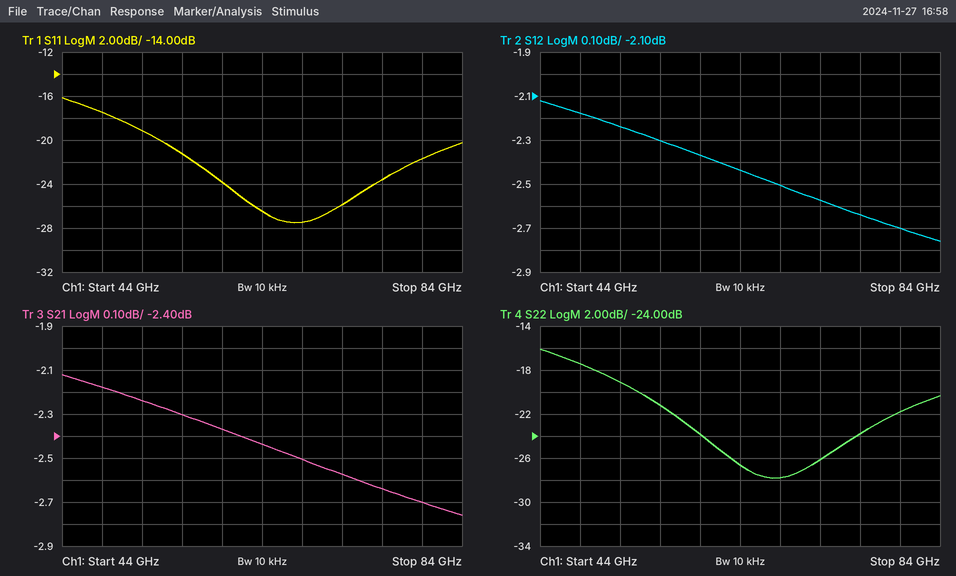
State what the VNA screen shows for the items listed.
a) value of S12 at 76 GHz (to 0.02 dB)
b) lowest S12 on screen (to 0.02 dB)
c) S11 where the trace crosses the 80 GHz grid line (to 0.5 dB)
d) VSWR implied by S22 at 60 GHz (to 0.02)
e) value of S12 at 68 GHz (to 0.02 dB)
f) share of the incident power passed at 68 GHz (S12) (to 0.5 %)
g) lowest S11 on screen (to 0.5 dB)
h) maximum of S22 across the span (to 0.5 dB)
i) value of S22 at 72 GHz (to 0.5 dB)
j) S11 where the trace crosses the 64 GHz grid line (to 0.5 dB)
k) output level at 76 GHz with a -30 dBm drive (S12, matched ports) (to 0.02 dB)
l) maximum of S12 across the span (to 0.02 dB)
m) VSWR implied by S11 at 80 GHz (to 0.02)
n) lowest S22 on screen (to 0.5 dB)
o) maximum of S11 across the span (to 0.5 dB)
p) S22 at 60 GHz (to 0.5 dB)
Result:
-2.64 dB
-2.76 dB
-21.5 dB
1.14
-2.50 dB
56.0 %
-27.5 dB
-16.0 dB
-26.0 dB
-26.5 dB
-32.64 dBm
-2.12 dB
1.18
-28.0 dB
-16.0 dB
-24.0 dB
